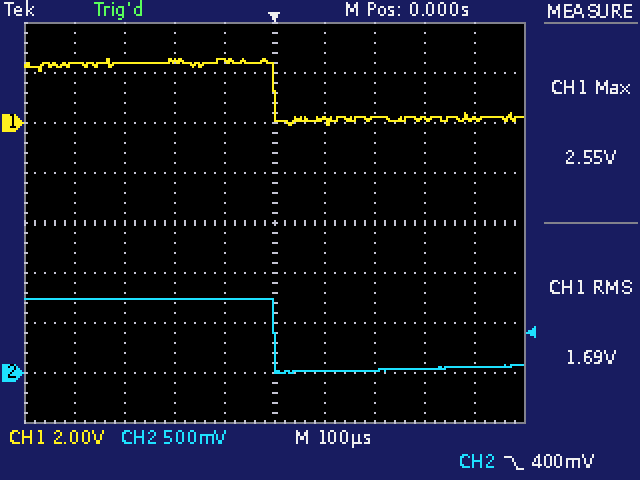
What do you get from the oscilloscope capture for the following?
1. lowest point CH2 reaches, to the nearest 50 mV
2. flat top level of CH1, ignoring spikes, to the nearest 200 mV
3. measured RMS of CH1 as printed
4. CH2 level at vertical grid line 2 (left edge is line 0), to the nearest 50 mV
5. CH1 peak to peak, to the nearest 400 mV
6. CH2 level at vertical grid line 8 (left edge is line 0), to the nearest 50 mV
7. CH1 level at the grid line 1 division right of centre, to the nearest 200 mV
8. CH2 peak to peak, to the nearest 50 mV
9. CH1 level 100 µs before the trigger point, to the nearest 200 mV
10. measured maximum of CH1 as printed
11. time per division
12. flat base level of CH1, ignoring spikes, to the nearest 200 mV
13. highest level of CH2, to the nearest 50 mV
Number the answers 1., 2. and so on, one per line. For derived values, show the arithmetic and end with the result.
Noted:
1. 0 mV
2. 2.4 V
3. 1.69 V
4. 750 mV
5. 2.8 V
6. 50 mV
7. 0.0 V
8. 750 mV − (0 mV) = 750 mV
9. 2.4 V
10. 2.55 V
11. 100 µs
12. 200 mV
13. 750 mV
